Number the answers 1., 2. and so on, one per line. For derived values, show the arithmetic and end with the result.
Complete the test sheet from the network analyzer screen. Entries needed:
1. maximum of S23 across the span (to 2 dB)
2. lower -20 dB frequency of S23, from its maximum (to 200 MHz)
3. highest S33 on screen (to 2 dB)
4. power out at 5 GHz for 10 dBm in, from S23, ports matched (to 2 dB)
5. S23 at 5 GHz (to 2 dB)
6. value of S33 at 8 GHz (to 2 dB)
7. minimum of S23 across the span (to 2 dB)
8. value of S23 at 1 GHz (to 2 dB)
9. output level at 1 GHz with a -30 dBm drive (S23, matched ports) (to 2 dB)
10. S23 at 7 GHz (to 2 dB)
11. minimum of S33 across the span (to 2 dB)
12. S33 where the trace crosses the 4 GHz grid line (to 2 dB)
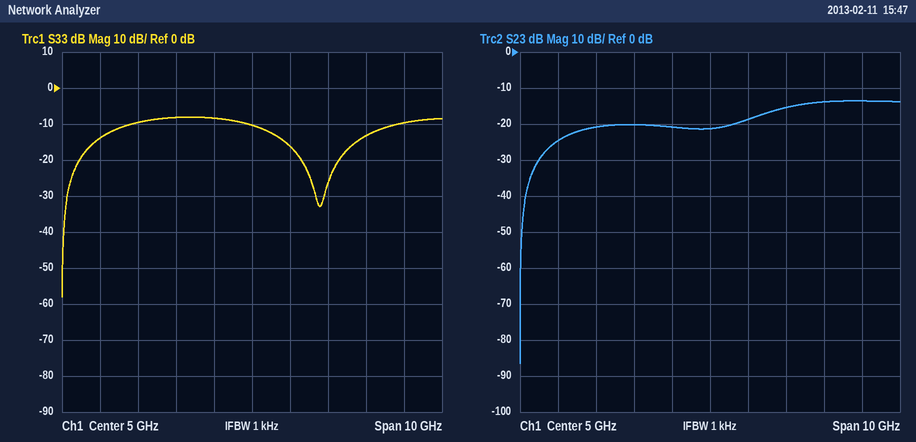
1. -14 dB
2. 400 MHz
3. -8 dB
4. 10 dBm + (-22 dB) = -12 dBm
5. -22 dB
6. -14 dB
7. -86 dB
8. -24 dB
9. -30 dBm + (-24 dB) = -54 dBm
10. -16 dB
11. -58 dB
12. -8 dB
